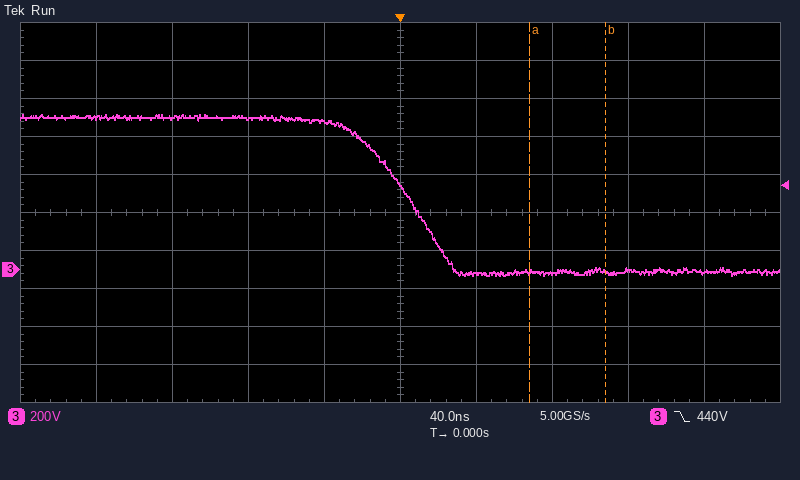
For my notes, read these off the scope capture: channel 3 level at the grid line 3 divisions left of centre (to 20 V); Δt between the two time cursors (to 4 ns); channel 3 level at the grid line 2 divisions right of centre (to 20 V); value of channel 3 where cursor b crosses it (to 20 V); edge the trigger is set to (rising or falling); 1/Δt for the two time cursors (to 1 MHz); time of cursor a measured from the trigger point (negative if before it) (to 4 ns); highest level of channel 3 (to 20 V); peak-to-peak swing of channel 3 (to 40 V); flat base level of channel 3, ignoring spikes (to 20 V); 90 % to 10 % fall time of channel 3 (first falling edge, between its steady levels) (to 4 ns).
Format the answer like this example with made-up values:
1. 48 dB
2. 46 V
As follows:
1. 800 V
2. 40 ns
3. -20 V
4. -20 V
5. falling
6. 25 MHz
7. +68 ns
8. 820 V
9. 840 V
10. -20 V
11. 48 ns
